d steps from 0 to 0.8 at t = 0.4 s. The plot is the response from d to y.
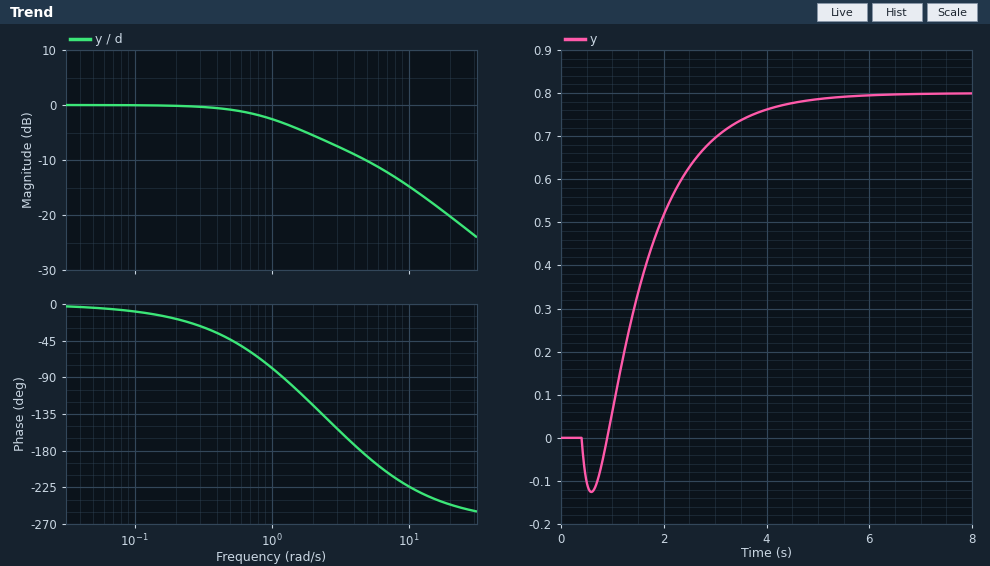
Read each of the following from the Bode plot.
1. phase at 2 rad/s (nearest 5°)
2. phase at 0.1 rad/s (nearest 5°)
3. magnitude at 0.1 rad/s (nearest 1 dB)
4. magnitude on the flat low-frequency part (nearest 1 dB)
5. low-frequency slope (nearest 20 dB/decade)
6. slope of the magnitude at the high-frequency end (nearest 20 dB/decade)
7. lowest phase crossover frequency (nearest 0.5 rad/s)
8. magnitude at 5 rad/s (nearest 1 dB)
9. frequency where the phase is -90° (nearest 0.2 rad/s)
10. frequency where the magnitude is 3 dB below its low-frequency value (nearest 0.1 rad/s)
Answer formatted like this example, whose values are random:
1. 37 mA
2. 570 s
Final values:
1. -125°
2. -10°
3. 0 dB
4. 0 dB
5. 0 dB/decade
6. -20 dB/decade
7. 4.5 rad/s
8. -10 dB
9. 1.2 rad/s
10. 1.1 rad/s
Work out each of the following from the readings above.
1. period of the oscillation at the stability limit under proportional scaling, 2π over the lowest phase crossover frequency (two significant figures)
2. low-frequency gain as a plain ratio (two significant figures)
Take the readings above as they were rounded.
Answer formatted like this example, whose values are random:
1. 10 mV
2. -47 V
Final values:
1. 1.4 s
2. 1.0
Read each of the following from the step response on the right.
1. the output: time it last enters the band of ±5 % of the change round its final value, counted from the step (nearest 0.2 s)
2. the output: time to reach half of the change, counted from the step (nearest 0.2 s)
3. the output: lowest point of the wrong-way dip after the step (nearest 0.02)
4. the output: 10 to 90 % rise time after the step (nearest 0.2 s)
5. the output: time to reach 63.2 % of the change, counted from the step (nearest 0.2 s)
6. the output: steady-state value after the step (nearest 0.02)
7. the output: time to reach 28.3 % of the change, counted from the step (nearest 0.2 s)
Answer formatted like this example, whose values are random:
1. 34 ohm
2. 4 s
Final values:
1. 3.6 s
2. 1.2 s
3. -0.12
4. 2.2 s
5. 1.6 s
6. 0.80
7. 0.8 s
